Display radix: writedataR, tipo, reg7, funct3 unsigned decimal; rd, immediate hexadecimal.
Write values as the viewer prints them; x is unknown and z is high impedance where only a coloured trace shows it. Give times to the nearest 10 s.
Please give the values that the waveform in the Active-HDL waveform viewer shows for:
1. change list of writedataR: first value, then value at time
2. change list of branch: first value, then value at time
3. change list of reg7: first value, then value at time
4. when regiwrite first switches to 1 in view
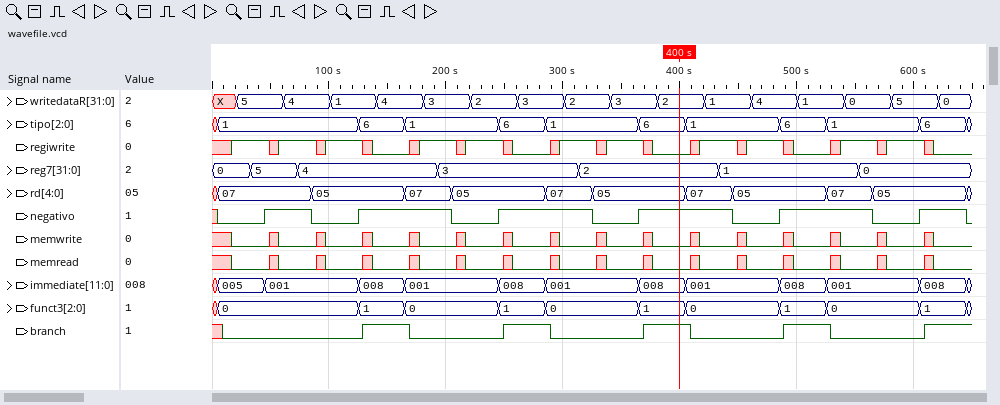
X, 5 at 20 s, 4 at 60 s, 1 at 100 s, 4 at 140 s, 3 at 180 s, 2 at 220 s, 3 at 260 s, 2 at 300 s, 3 at 340 s, 2 at 380 s, 1 at 420 s, 4 at 460 s, 1 at 500 s, 0 at 540 s, 5 at 580 s, 0 at 620 s
x, 0 at 10 s, 1 at 130 s, 0 at 170 s, 1 at 250 s, 0 at 290 s, 1 at 370 s, 0 at 410 s, 1 at 490 s, 0 at 530 s, 1 at 610 s
0, 5 at 30 s, 4 at 70 s, 3 at 190 s, 2 at 310 s, 1 at 430 s, 0 at 550 s
20 s
